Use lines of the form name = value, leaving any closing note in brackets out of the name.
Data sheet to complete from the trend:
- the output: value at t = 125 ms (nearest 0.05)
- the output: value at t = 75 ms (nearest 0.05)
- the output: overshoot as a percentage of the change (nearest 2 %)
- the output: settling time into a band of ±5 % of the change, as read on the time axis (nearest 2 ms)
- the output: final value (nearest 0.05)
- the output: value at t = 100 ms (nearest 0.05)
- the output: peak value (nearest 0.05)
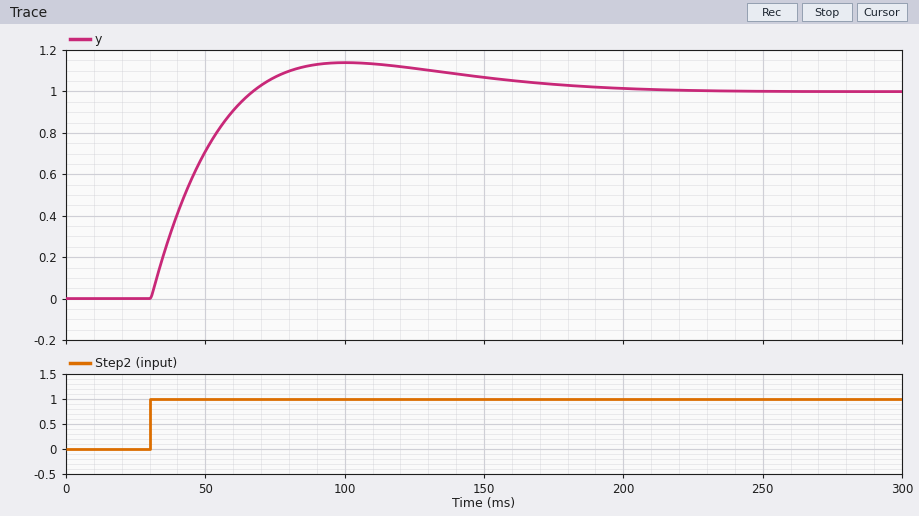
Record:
the output: value at t = 125 ms = 1.10
the output: value at t = 75 ms = 1.05
the output: overshoot as a percentage of the change = 14 %
the output: settling time into a band of ±5 % of the change, as read on the time axis = 162 ms
the output: final value = 1.00
the output: value at t = 100 ms = 1.15
the output: peak value = 1.15
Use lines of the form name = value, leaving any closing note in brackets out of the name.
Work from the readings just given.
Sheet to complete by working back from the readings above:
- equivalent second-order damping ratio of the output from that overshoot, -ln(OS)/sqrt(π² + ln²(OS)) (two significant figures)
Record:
equivalent second-order damping ratio of the output from that overshoot, -ln(OS)/sqrt(π² + ln²(OS)) = 0.53
